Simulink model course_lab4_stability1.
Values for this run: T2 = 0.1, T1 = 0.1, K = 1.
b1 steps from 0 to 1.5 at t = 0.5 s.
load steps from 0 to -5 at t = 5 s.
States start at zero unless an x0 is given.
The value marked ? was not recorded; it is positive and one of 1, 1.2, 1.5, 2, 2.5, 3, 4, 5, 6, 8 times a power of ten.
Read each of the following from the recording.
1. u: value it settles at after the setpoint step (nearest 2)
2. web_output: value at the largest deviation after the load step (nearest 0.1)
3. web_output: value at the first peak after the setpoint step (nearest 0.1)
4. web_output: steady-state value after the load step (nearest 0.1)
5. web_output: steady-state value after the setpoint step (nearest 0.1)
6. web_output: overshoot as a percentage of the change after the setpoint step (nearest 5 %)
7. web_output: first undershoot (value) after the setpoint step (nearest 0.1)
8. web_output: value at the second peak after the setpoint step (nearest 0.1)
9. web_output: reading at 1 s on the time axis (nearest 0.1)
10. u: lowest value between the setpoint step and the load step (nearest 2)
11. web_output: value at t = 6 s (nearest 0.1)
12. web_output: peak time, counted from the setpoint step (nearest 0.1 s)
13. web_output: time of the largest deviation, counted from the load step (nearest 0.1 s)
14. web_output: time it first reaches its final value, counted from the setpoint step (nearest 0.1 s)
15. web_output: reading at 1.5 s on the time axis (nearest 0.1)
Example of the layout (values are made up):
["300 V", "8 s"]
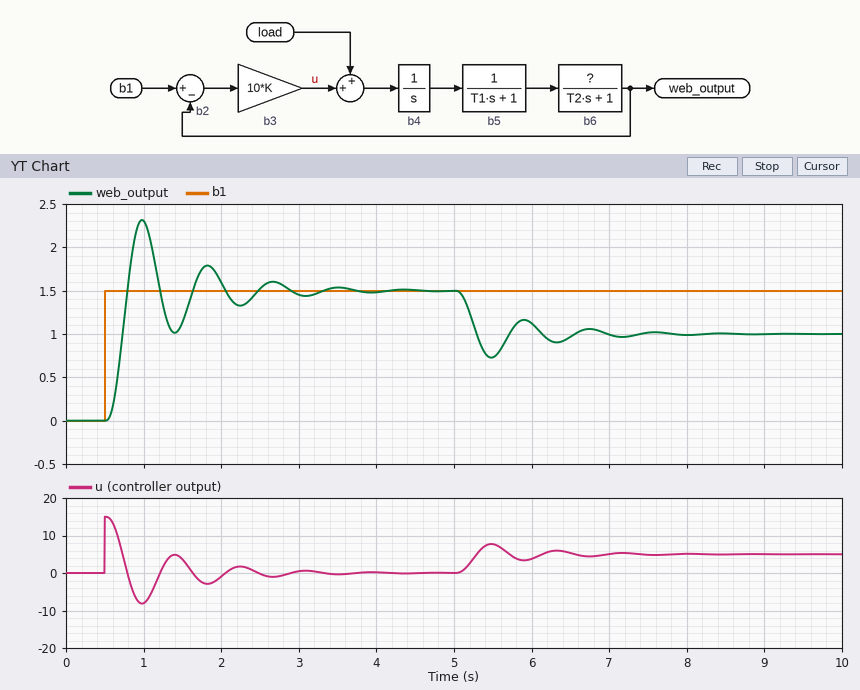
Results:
["0", "0.7", "2.3", "1.0", "1.5", "55 %", "1.0", "1.8", "2.3", "-8", "1.1", "0.5 s", "0.5 s", "0.3 s", "1.1"]
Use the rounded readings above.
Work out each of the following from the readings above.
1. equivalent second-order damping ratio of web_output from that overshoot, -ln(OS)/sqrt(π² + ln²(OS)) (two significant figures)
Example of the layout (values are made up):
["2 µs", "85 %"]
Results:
["0.19"]
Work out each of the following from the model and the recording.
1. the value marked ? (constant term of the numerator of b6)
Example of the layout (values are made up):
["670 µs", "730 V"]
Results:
["1"]
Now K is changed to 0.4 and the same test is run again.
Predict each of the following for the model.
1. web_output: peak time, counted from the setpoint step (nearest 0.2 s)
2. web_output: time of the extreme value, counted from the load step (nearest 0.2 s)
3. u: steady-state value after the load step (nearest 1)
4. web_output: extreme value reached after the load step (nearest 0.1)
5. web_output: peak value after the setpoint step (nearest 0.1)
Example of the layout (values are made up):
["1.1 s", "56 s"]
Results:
["0.8 s", "0.8 s", "5", "0.0", "1.8"]
